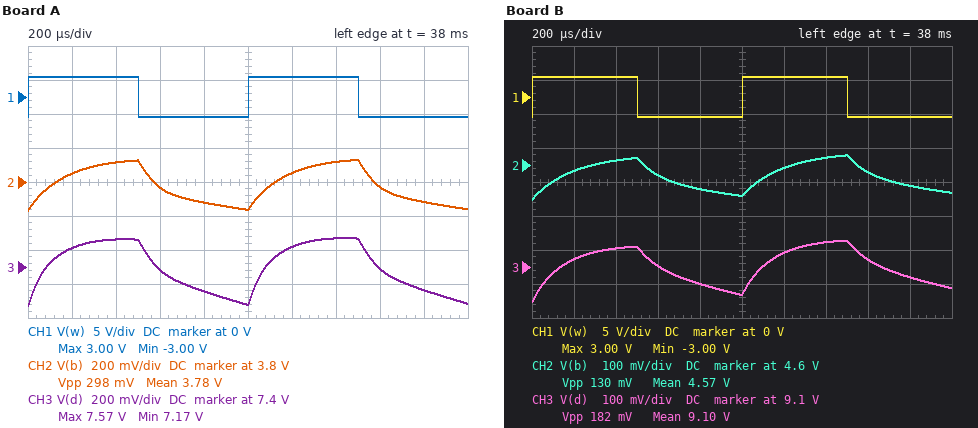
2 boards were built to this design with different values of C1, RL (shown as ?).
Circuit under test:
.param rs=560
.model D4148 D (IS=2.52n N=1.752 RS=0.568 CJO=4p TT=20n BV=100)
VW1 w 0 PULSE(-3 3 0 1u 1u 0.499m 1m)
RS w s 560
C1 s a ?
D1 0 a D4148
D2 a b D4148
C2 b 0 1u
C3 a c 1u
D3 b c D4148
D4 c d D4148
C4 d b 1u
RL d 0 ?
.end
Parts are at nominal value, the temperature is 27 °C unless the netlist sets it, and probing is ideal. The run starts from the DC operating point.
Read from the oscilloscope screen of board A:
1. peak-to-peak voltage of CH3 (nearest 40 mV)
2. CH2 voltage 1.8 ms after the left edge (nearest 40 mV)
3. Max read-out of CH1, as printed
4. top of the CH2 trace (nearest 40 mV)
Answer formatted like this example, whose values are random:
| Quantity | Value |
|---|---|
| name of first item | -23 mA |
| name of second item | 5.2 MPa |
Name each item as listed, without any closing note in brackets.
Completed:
| Quantity | Value |
|---|---|
| peak-to-peak voltage of CH3 | 400 mV |
| CH2 voltage 1.8 ms after the left edge | 3.68 V |
| Max read-out of CH1, as printed | 3.00 V |
| top of the CH2 trace | 3.92 V |
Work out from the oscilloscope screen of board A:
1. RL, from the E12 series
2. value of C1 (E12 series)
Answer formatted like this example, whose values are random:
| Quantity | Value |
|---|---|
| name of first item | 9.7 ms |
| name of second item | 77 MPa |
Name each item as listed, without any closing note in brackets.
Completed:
| Quantity | Value |
|---|---|
| RL, from the E12 series | 39 kΩ |
| value of C1 | 560 nF |
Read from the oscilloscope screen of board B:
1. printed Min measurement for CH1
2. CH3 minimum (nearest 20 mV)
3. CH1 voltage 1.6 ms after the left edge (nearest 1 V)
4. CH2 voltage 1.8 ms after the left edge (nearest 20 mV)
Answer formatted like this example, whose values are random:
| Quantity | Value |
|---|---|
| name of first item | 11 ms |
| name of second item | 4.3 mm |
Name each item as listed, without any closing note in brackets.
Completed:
| Quantity | Value |
|---|---|
| printed Min measurement for CH1 | -3.00 V |
| CH3 minimum | 9.00 V |
| CH1 voltage 1.6 ms after the left edge | -3 V |
| CH2 voltage 1.8 ms after the left edge | 4.54 V |
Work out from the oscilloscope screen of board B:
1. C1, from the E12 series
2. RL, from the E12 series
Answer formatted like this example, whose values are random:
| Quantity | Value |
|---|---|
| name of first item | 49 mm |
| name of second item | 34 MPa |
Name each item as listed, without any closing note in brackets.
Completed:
| Quantity | Value |
|---|---|
| C1, from the E12 series | 560 nF |
| RL, from the E12 series | 150 kΩ |
